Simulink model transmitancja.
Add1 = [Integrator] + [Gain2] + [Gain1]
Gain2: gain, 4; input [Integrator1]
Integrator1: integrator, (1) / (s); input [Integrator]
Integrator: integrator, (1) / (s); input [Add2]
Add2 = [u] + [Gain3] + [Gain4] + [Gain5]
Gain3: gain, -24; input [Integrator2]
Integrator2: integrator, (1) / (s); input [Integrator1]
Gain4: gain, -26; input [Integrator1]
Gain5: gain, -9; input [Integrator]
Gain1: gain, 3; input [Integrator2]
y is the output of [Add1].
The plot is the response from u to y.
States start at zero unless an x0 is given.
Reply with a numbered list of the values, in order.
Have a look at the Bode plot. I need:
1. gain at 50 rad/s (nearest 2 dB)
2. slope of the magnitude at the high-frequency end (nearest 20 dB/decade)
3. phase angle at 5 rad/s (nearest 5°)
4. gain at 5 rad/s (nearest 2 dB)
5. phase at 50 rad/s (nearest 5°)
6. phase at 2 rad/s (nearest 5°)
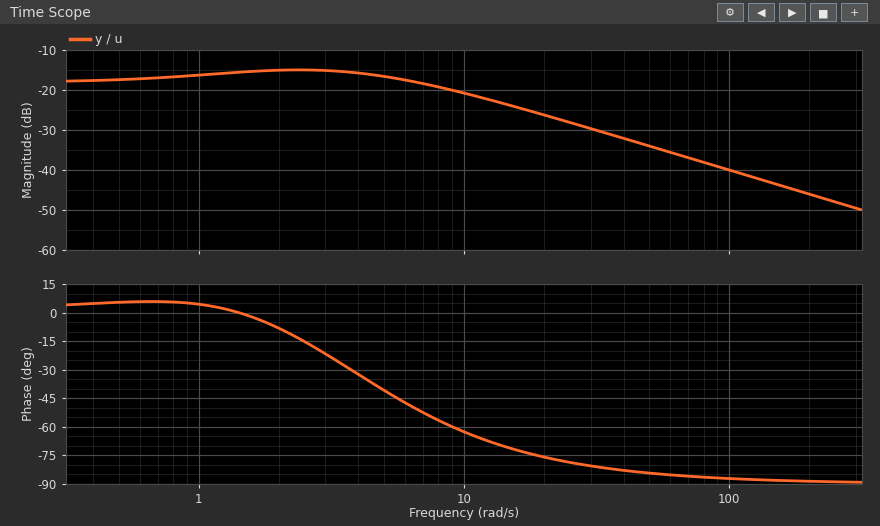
1. -34 dB
2. -20 dB/decade
3. -40°
4. -16 dB
5. -85°
6. -10°
